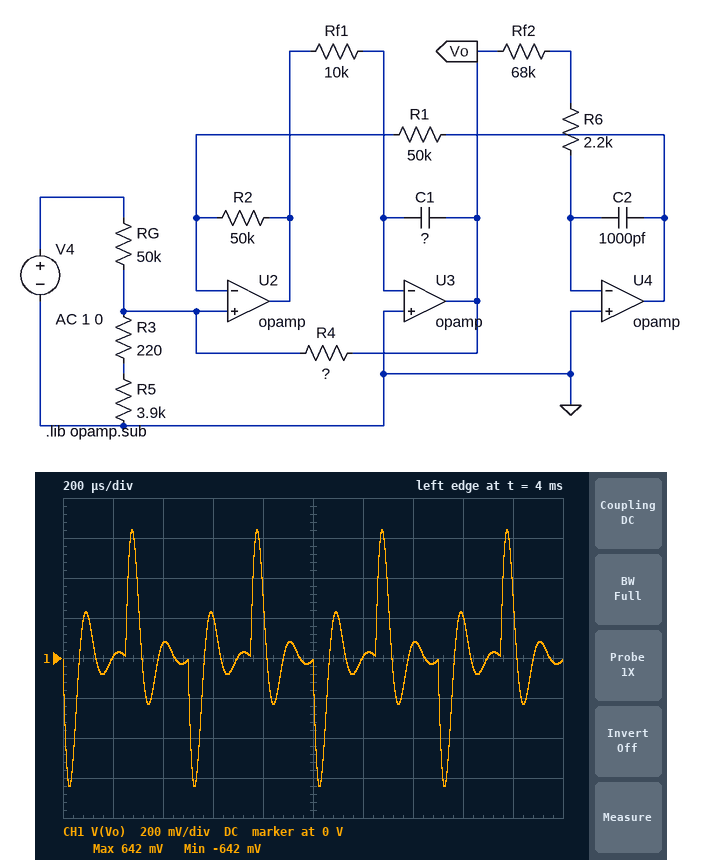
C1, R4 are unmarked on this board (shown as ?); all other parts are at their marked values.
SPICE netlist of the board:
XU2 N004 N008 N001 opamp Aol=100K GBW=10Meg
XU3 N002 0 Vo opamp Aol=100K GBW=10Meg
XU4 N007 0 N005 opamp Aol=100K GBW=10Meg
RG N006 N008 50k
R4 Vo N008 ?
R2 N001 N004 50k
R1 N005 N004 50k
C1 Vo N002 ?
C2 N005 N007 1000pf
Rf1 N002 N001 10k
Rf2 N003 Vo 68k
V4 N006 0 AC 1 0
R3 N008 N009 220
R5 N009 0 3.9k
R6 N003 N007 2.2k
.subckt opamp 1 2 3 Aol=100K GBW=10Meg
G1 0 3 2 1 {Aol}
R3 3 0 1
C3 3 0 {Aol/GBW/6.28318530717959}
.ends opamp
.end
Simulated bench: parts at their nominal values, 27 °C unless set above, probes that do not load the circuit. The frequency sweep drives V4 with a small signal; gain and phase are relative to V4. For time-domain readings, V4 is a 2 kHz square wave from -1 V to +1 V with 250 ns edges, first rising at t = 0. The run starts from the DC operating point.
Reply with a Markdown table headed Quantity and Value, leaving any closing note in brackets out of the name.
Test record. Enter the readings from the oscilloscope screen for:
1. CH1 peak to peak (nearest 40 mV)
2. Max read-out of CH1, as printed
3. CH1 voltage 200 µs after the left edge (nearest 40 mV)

| Quantity | Value |
|---|---|
| CH1 peak to peak | 1.28 V |
| Max read-out of CH1, as printed | 642 mV |
| CH1 voltage 200 µs after the left edge | 0 V |
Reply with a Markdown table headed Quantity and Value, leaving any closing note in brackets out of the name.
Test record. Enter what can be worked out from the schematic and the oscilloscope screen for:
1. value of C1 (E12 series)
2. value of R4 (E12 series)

| Quantity | Value |
|---|---|
| value of C1 | 560 pF |
| value of R4 | 39 kΩ |
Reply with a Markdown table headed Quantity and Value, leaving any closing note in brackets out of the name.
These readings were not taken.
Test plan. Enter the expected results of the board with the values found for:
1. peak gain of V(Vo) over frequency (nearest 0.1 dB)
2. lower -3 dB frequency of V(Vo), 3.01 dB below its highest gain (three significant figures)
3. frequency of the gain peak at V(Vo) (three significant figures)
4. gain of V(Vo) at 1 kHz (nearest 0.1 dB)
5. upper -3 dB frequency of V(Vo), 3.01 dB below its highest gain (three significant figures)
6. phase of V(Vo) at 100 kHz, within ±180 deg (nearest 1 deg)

| Quantity | Value |
|---|---|
| peak gain of V(Vo) over frequency | -2.1 dB |
| lower -3 dB frequency of V(Vo), 3.01 dB below its highest gain | 5.89 kHz |
| frequency of the gain peak at V(Vo) | 8.02 kHz |
| gain of V(Vo) at 1 kHz | -24.2 dB |
| upper -3 dB frequency of V(Vo), 3.01 dB below its highest gain | 10.9 kHz |
| phase of V(Vo) at 100 kHz, within ±180 deg | 91 deg |
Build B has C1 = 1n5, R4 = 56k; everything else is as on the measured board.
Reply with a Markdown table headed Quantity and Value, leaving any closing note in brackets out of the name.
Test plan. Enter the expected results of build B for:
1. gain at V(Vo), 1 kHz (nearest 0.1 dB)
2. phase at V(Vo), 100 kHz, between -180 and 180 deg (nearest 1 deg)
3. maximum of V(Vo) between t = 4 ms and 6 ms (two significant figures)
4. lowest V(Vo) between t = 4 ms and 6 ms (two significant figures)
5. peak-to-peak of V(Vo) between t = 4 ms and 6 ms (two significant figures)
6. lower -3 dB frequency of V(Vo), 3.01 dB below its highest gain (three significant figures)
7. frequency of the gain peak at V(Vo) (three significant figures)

| Quantity | Value |
|---|---|
| gain at V(Vo), 1 kHz | -23.7 dB |
| phase at V(Vo), 100 kHz, between -180 and 180 deg | 89 deg |
| maximum of V(Vo) between t = 4 ms and 6 ms | 430 mV |
| lowest V(Vo) between t = 4 ms and 6 ms | -430 mV |
| peak-to-peak of V(Vo) between t = 4 ms and 6 ms | 860 mV |
| lower -3 dB frequency of V(Vo), 3.01 dB below its highest gain | 4.28 kHz |
| frequency of the gain peak at V(Vo) | 4.90 kHz |
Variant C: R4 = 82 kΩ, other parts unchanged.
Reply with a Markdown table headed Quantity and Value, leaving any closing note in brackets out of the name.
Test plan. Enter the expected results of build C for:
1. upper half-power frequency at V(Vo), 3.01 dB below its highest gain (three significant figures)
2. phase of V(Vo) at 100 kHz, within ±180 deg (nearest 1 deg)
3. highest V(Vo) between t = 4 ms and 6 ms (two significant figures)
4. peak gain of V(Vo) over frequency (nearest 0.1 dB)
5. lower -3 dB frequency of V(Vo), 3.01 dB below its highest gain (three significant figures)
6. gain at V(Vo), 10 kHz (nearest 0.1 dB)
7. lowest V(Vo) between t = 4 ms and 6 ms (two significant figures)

| Quantity | Value |
|---|---|
| upper half-power frequency at V(Vo), 3.01 dB below its highest gain | 9.36 kHz |
| phase of V(Vo) at 100 kHz, within ±180 deg | 90 deg |
| highest V(Vo) between t = 4 ms and 6 ms | 720 mV |
| peak gain of V(Vo) over frequency | 4.4 dB |
| lower -3 dB frequency of V(Vo), 3.01 dB below its highest gain | 6.87 kHz |
| gain at V(Vo), 10 kHz | -0.5 dB |
| lowest V(Vo) between t = 4 ms and 6 ms | -720 mV |
